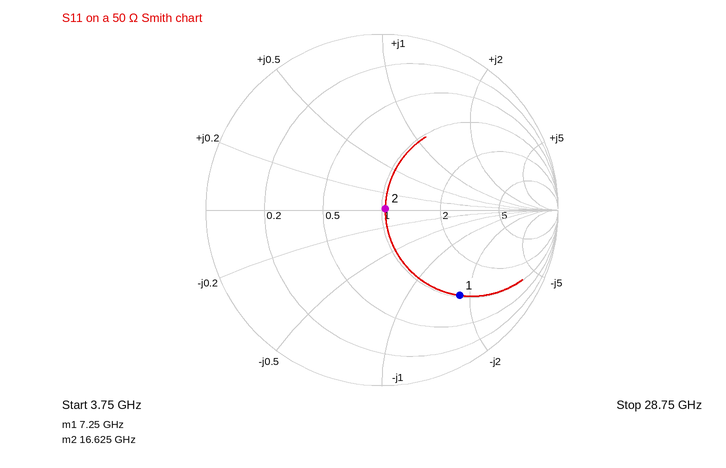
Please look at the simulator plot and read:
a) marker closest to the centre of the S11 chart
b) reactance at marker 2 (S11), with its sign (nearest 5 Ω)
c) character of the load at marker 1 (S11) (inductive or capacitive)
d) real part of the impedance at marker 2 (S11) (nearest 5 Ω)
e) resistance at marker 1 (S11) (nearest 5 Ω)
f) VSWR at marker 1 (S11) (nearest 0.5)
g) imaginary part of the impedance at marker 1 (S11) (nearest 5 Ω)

marker 2
0 Ω
capacitive
50 Ω
50 Ω
5.0
-90 Ω
